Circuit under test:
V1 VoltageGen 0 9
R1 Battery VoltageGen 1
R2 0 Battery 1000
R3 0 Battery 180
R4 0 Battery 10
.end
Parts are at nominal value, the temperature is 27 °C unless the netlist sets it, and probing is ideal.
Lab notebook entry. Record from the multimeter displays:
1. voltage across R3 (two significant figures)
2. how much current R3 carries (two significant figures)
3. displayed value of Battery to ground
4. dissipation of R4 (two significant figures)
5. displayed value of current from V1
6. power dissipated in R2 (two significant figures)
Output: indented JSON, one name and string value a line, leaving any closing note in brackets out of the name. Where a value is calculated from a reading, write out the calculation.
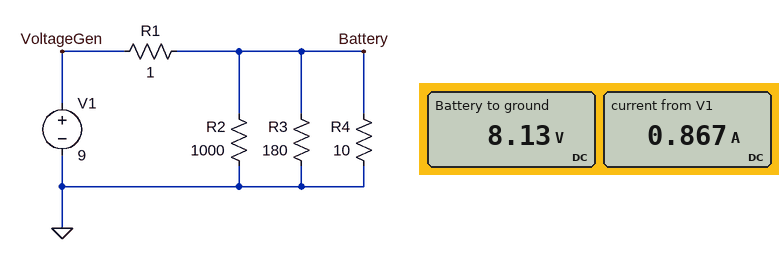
{
  "voltage across R3": "8.13 V = 8.1 V",
  "how much current R3 carries": "(8.13 V) / 180 Ω = 45 mA",
  "displayed value of Battery to ground": "8.13 V",
  "dissipation of R4": "(8.13 V)^2 / 10 Ω = 6.6 W",
  "displayed value of current from V1": "0.867 A",
  "power dissipated in R2": "(8.13 V)^2 / 1 kΩ = 66 mW"
}
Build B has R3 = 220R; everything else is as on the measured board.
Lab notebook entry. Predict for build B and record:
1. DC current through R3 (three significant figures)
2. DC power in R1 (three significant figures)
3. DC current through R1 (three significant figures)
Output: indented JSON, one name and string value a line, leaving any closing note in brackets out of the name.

{
  "DC current through R3": "37.0 mA",
  "DC power in R1": "738 mW",
  "DC current through R1": "859 mA"
}
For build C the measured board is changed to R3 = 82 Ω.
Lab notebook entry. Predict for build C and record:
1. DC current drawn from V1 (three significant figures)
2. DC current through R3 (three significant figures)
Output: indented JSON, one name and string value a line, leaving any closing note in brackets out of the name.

{
  "DC current drawn from V1": "915 mA",
  "DC current through R3": "98.6 mA"
}
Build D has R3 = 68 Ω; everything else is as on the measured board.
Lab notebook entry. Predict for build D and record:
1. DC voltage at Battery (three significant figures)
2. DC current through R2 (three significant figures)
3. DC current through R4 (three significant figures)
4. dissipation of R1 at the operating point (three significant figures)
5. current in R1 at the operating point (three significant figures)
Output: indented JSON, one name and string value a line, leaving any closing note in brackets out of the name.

{
  "DC voltage at Battery": "8.07 V",
  "DC current through R2": "8.07 mA",
  "DC current through R4": "807 mA",
  "dissipation of R1 at the operating point": "871 mW",
  "current in R1 at the operating point": "933 mA"
}
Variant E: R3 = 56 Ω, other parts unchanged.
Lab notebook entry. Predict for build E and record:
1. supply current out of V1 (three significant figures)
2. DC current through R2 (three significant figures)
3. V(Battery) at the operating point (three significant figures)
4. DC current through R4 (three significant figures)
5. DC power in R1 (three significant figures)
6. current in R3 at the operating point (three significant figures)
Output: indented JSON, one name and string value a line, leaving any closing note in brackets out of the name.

{
  "supply current out of V1": "956 mA",
  "DC current through R2": "8.04 mA",
  "V(Battery) at the operating point": "8.04 V",
  "DC current through R4": "804 mA",
  "DC power in R1": "914 mW",
  "current in R3 at the operating point": "144 mA"
}
